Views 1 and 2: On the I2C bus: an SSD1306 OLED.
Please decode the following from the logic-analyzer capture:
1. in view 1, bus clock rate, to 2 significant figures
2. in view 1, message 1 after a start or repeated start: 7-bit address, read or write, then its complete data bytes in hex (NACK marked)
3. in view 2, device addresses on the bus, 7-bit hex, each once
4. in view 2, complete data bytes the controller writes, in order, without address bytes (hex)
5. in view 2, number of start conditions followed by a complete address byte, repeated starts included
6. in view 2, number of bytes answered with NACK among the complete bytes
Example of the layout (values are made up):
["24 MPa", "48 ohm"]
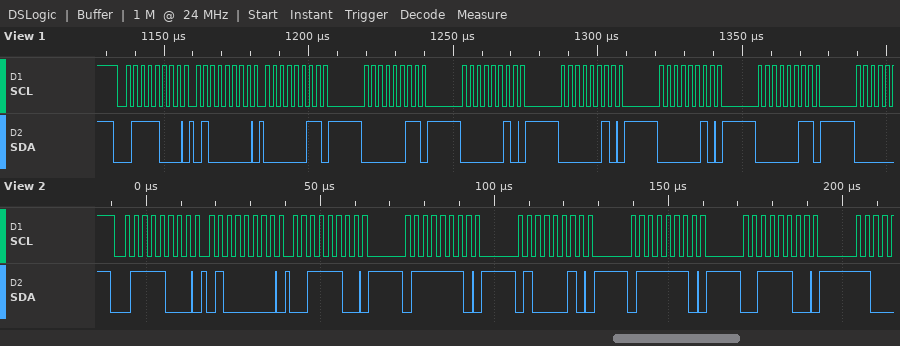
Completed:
["400 kHz", "0x3C write: 40 03 03 02 02 02 03", "0x3C", "40 3C 7E 42 7E 3C", "1", "0"]
